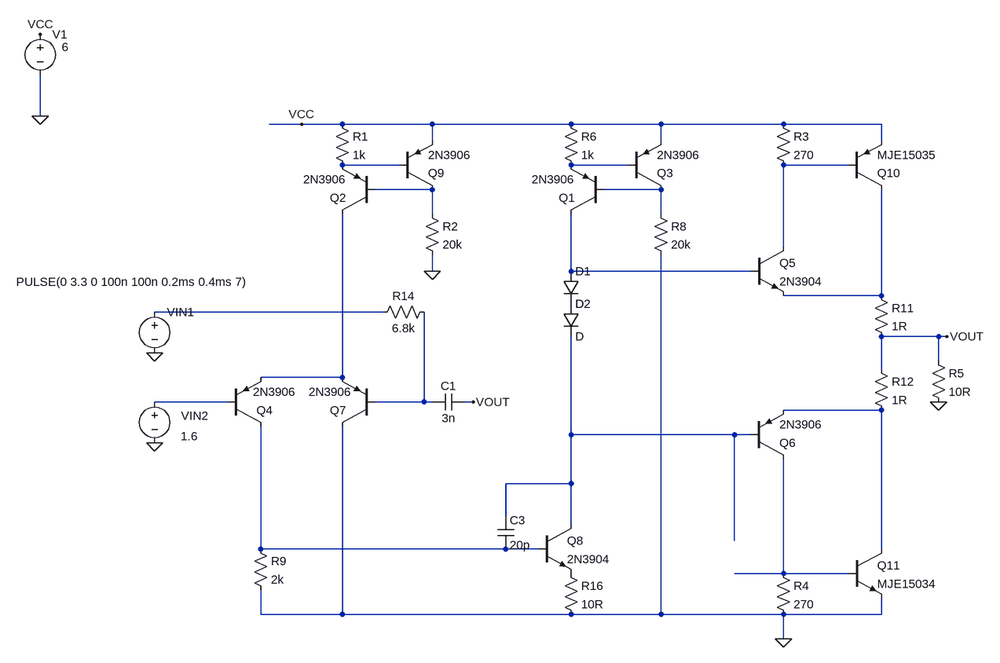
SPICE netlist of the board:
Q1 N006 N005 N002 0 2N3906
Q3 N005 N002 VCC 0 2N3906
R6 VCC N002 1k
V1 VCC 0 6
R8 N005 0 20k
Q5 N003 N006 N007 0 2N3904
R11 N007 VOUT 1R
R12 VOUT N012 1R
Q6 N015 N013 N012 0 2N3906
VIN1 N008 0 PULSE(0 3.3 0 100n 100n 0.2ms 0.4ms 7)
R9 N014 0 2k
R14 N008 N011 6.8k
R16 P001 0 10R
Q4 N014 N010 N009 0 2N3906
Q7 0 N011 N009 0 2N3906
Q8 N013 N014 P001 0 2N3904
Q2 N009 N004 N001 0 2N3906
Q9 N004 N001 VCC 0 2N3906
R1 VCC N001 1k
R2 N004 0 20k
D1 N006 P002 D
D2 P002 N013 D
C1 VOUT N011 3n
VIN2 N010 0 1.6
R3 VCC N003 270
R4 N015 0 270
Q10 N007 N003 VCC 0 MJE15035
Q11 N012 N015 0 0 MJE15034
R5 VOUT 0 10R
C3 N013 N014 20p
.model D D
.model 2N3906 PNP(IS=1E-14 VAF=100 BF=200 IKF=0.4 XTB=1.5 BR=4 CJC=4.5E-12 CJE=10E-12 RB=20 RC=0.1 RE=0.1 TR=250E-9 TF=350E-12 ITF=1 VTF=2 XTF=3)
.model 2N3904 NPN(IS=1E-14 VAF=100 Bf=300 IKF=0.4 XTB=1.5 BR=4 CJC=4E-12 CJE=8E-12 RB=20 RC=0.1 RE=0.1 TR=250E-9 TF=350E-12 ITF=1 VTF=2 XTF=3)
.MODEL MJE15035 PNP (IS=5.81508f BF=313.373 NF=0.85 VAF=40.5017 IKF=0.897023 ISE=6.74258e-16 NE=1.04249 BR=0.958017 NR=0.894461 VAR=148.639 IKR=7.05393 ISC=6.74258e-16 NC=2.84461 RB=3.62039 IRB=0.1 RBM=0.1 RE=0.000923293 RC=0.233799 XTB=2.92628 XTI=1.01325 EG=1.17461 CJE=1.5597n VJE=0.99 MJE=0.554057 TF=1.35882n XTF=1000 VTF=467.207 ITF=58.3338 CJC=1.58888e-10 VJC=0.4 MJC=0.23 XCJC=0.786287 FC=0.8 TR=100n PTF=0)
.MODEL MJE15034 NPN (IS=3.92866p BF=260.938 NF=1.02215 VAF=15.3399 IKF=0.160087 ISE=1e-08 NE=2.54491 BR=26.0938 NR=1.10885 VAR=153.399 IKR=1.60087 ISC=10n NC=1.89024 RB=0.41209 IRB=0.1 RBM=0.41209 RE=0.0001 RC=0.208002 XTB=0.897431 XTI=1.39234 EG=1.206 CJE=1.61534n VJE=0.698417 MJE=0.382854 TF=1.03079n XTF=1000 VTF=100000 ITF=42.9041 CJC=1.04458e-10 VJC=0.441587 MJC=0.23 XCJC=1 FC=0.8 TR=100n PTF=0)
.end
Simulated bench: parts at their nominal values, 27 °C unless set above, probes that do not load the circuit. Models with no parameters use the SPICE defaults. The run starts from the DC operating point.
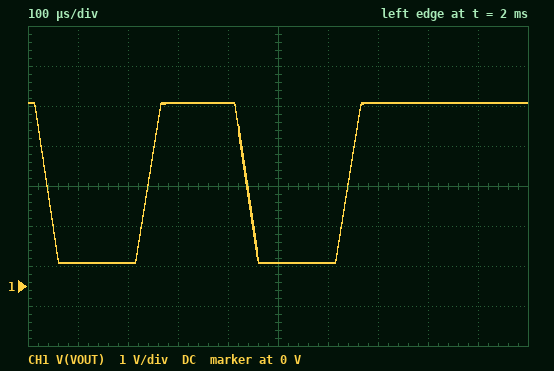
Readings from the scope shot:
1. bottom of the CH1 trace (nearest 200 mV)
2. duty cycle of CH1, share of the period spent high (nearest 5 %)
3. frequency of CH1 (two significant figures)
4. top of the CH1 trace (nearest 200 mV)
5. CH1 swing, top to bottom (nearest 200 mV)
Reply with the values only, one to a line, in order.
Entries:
600 mV
50 %
2.5 kHz
4.6 V
4.0 V
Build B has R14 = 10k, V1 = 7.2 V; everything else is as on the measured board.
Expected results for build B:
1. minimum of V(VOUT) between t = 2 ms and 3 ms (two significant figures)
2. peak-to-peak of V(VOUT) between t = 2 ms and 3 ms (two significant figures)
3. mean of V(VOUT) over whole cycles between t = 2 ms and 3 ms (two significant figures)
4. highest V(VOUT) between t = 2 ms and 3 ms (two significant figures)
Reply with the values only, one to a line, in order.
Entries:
570 mV
5.0 V
3.0 V
5.6 V
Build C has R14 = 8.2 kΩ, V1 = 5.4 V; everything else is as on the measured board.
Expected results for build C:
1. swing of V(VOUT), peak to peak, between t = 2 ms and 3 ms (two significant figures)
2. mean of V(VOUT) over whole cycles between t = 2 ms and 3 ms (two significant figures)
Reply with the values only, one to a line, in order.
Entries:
3.5 V
2.3 V
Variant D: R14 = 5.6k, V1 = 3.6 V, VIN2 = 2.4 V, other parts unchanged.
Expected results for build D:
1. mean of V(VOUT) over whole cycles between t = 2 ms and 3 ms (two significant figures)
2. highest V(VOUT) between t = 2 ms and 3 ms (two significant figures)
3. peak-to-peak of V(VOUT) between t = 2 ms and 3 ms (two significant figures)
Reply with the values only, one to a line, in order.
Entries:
1.7 V
2.5 V
1.9 V
